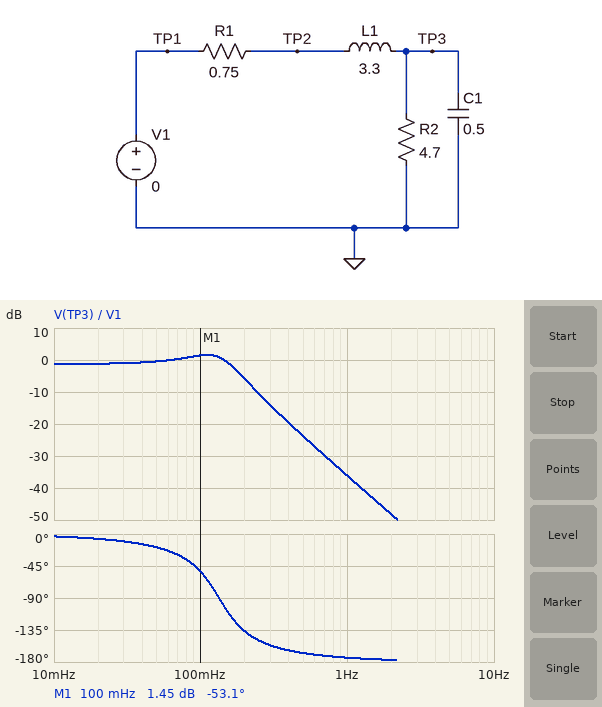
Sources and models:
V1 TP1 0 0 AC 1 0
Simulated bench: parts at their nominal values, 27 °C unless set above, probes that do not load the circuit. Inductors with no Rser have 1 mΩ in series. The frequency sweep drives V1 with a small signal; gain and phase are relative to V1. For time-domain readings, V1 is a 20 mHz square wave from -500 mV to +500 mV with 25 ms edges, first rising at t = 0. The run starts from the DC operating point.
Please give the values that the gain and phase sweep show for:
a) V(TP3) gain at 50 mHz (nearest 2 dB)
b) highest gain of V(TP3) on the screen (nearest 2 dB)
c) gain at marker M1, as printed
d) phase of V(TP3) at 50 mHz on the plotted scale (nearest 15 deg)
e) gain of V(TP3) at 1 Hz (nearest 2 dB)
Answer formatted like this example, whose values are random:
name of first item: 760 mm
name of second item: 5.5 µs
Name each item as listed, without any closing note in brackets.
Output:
V(TP3) gain at 50 mHz: 0 dB
highest gain of V(TP3) on the screen: 2 dB
gain at marker M1, as printed: 1.45 dB
phase of V(TP3) at 50 mHz on the plotted scale: -15 deg
gain of V(TP3) at 1 Hz: -36 dB
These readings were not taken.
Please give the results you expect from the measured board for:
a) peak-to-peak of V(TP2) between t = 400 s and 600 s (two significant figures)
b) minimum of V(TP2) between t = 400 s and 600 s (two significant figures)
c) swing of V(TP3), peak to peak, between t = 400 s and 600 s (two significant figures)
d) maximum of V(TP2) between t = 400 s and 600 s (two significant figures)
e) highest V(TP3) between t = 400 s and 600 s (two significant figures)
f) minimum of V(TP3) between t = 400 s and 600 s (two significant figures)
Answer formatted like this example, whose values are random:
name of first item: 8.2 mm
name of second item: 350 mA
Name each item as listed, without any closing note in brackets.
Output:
peak-to-peak of V(TP2) between t = 400 s and 600 s: 1.1 V
minimum of V(TP2) between t = 400 s and 600 s: -570 mV
swing of V(TP3), peak to peak, between t = 400 s and 600 s: 1.3 V
maximum of V(TP2) between t = 400 s and 600 s: 570 mV
highest V(TP3) between t = 400 s and 600 s: 660 mV
minimum of V(TP3) between t = 400 s and 600 s: -660 mV
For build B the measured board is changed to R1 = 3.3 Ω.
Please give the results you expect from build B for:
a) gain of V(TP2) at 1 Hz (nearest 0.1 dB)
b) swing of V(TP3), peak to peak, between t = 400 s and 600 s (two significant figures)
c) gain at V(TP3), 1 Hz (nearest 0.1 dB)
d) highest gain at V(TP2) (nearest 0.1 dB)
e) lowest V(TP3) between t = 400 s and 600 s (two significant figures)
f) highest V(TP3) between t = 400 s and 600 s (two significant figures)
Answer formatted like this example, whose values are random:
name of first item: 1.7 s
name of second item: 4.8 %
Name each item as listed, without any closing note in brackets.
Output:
gain of V(TP2) at 1 Hz: -0.1 dB
swing of V(TP3), peak to peak, between t = 400 s and 600 s: 640 mV
gain at V(TP3), 1 Hz: -36.3 dB
highest gain at V(TP2): 0 dB
lowest V(TP3) between t = 400 s and 600 s: -320 mV
highest V(TP3) between t = 400 s and 600 s: 320 mV
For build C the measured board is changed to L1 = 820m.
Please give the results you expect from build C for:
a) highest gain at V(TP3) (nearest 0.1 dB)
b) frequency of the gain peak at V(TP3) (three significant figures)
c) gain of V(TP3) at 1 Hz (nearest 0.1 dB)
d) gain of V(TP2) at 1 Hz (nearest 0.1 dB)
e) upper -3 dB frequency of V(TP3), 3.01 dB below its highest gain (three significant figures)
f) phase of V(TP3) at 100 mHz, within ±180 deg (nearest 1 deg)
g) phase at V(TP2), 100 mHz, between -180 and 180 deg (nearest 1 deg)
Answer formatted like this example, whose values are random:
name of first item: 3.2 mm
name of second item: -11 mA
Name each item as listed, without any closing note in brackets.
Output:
highest gain at V(TP3): 1.4 dB
frequency of the gain peak at V(TP3): 221 mHz
gain of V(TP3) at 1 Hz: -23.8 dB
gain of V(TP2) at 1 Hz: -0.1 dB
upper -3 dB frequency of V(TP3), 3.01 dB below its highest gain: 318 mHz
phase of V(TP3) at 100 mHz, within ±180 deg: -19 deg
phase at V(TP2), 100 mHz, between -180 and 180 deg: -12 deg
